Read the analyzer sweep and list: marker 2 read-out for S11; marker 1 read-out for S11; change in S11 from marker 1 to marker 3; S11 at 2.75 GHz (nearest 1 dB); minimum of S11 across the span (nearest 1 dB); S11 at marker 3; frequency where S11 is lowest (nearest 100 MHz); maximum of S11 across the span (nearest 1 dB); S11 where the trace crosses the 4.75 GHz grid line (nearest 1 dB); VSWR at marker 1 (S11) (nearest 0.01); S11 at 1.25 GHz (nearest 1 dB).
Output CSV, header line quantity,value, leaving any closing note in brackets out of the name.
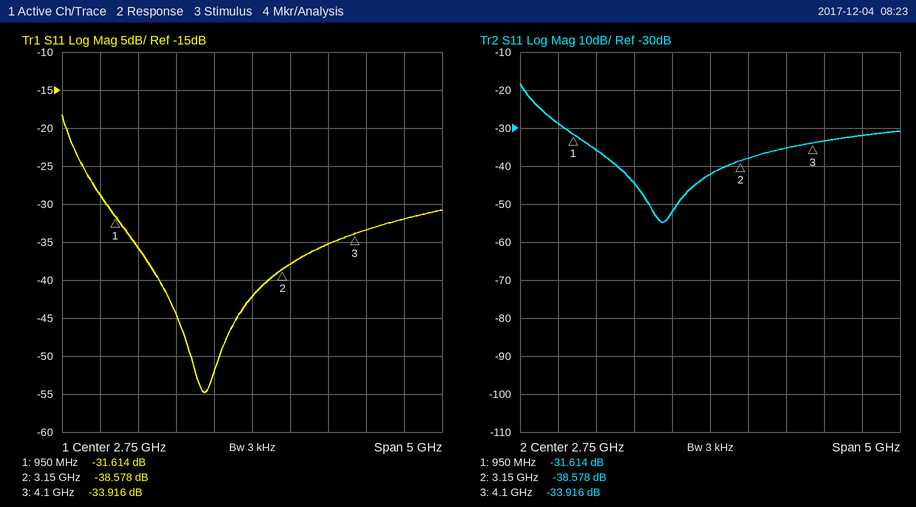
quantity,value
marker 2 read-out for S11,-38.578 dB
marker 1 read-out for S11,-31.614 dB
change in S11 from marker 1 to marker 3,-2.302 dB
S11 at 2.75 GHz,-42 dB
minimum of S11 across the span,-55 dB
S11 at marker 3,-33.916 dB
frequency where S11 is lowest,2.1 GHz
maximum of S11 across the span,-18 dB
S11 where the trace crosses the 4.75 GHz grid line,-32 dB
VSWR at marker 1 (S11),1.05
S11 at 1.25 GHz,-36 dB
